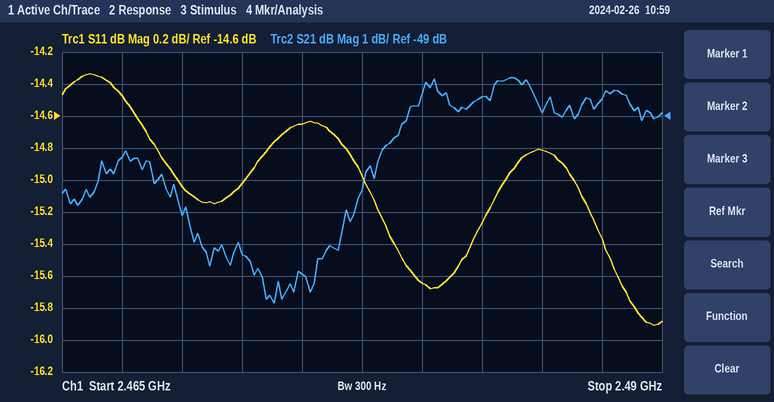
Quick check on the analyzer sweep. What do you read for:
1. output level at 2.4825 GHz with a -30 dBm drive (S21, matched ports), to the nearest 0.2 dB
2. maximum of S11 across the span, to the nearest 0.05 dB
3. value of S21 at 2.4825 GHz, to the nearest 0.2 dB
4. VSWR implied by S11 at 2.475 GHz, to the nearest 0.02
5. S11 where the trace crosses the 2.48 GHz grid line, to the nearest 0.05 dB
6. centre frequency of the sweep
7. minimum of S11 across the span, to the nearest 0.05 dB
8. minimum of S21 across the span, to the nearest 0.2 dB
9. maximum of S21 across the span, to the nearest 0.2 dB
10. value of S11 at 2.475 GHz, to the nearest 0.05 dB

-78.4 dBm
-14.35 dB
-48.4 dB
1.46
-15.65 dB
2.4775 GHz
-15.90 dB
-54.8 dB
-47.8 dB
-14.65 dB
